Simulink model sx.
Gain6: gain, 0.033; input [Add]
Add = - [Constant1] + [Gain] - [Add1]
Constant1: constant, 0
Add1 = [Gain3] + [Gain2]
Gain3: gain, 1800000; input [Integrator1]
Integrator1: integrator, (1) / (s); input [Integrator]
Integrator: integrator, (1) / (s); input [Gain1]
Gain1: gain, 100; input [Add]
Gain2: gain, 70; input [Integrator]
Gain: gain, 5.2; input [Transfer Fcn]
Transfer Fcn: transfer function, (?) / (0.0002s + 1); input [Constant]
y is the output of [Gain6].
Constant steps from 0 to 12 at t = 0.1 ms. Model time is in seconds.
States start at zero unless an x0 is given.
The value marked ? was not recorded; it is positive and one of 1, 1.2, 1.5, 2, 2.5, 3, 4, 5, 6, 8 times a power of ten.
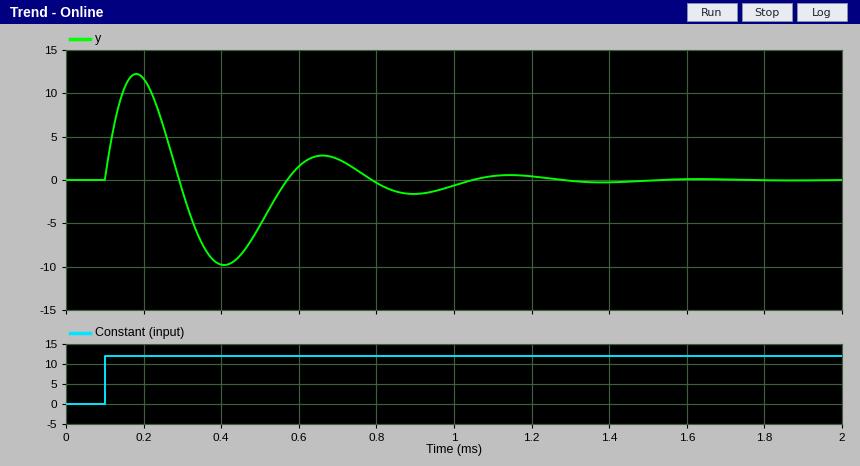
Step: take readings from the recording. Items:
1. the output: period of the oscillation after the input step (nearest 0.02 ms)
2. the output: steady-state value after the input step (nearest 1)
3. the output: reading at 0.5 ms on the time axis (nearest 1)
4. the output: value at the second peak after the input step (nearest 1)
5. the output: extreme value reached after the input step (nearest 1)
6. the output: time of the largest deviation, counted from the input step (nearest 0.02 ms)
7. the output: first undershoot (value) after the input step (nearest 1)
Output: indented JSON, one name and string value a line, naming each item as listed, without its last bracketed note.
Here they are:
{
  "the output: period of the oscillation after the input step": "0.48 ms",
  "the output: steady-state value after the input step": "0",
  "the output: reading at 0.5 ms on the time axis": "-5",
  "the output: value at the second peak after the input step": "3",
  "the output: extreme value reached after the input step": "12",
  "the output: time of the largest deviation, counted from the input step": "0.08 ms",
  "the output: first undershoot (value) after the input step": "-10"
}
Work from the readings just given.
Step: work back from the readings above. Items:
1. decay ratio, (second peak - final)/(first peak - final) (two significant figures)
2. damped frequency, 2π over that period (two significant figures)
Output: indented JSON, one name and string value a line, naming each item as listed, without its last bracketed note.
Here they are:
{
  "decay ratio, (second peak - final)/(first peak - final)": "0.25",
  "damped frequency, 2π over that period": "13 rad/ms"
}
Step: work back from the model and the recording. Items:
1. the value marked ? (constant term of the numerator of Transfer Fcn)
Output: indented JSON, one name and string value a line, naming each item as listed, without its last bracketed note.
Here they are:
{
  "the value marked ?": "30"
}
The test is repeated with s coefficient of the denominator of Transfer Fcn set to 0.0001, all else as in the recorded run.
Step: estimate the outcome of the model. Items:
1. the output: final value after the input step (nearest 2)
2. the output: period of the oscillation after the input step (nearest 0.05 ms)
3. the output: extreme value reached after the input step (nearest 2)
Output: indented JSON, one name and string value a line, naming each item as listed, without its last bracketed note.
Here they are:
{
  "the output: final value after the input step": "0",
  "the output: period of the oscillation after the input step": "0.45 ms",
  "the output: extreme value reached after the input step": "20"
}
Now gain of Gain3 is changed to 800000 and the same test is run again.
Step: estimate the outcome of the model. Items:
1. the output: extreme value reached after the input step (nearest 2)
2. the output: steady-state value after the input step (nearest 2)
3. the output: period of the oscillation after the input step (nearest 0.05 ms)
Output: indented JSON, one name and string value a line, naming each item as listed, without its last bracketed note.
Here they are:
{
  "the output: extreme value reached after the input step": "14",
  "the output: steady-state value after the input step": "0",
  "the output: period of the oscillation after the input step": "0.75 ms"
}
